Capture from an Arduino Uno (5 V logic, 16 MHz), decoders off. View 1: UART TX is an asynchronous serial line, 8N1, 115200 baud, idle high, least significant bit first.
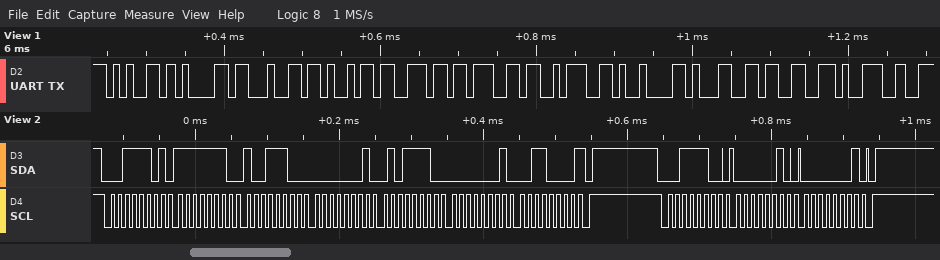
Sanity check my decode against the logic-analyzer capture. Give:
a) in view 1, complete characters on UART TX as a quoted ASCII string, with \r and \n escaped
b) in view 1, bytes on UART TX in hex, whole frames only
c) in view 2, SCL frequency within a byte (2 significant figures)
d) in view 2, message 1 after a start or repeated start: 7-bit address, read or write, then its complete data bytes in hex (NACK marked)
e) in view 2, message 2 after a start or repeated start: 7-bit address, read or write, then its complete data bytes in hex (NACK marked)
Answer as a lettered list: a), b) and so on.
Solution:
a) "eading:\t139"
b) 65 61 64 69 6E 67 3A 09 31 33 39
c) 100 kHz
d) 0x1E read: FE 9C 01 5E 01 30 NACK
e) 0x1E write: 02 01
